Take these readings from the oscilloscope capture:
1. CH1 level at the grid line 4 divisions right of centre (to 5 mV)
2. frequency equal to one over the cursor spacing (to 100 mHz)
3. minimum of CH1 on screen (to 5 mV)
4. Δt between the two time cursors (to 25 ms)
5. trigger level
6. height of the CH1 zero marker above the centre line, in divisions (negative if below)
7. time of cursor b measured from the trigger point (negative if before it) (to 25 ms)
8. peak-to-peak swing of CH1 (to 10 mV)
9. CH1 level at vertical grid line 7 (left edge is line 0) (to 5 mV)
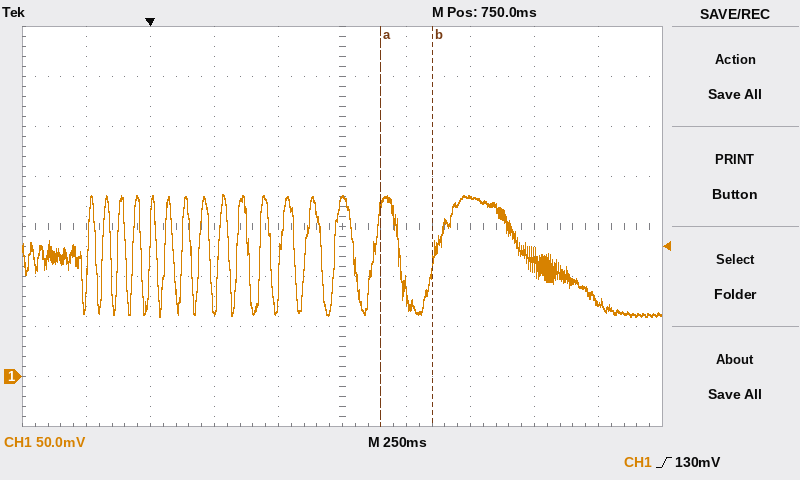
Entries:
75 mV
5.0 Hz
60 mV
200 ms
130 mV
-3.0 div
+1.100 s
120 mV
180 mV
